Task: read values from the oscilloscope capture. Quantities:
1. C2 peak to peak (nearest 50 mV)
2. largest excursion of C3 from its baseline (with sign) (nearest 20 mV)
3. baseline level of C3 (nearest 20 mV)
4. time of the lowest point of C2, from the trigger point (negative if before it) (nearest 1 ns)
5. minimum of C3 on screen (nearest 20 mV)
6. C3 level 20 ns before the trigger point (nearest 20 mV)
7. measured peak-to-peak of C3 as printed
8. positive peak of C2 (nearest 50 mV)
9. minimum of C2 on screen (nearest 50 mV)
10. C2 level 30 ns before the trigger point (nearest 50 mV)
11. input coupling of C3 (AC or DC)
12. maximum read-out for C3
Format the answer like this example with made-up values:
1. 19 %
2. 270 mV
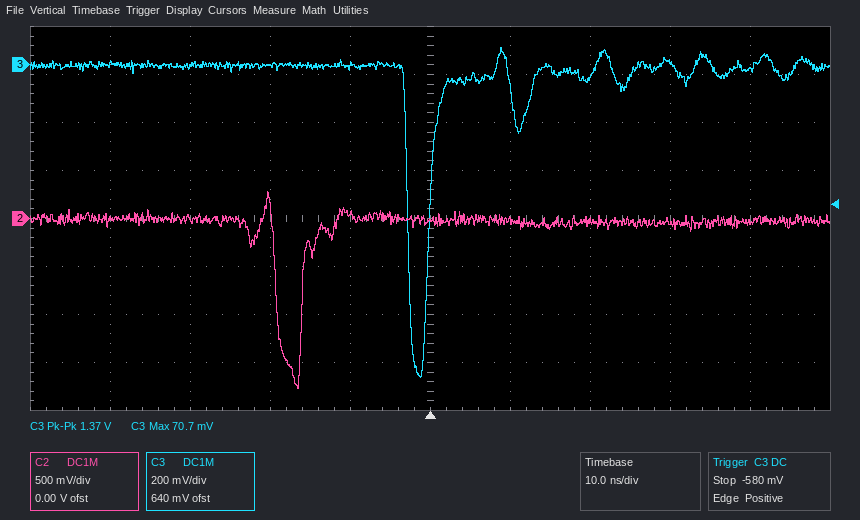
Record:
1. 2.05 V
2. -1.30 V
3. 0 mV
4. -17 ns
5. -1.30 V
6. 0 mV
7. 1.37 V
8. 300 mV
9. -1.75 V
10. 0 mV
11. DC
12. 70.7 mV
